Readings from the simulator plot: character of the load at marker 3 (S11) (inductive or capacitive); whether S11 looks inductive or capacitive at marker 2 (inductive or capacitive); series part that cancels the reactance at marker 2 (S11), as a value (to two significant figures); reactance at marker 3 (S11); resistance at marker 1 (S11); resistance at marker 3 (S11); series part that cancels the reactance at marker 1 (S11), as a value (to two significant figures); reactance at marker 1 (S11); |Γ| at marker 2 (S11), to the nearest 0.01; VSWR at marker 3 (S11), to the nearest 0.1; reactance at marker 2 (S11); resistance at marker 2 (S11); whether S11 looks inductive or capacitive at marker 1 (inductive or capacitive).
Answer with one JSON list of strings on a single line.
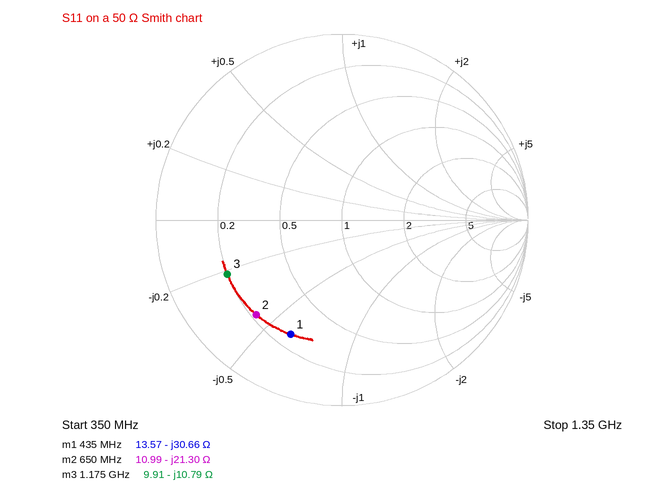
["capacitive", "capacitive", "5.2 nH", "-10.79 Ω", "13.57 Ω", "9.91 Ω", "11 nH", "-30.66 Ω", "0.69", "5.3", "-21.30 Ω", "10.99 Ω", "capacitive"]
